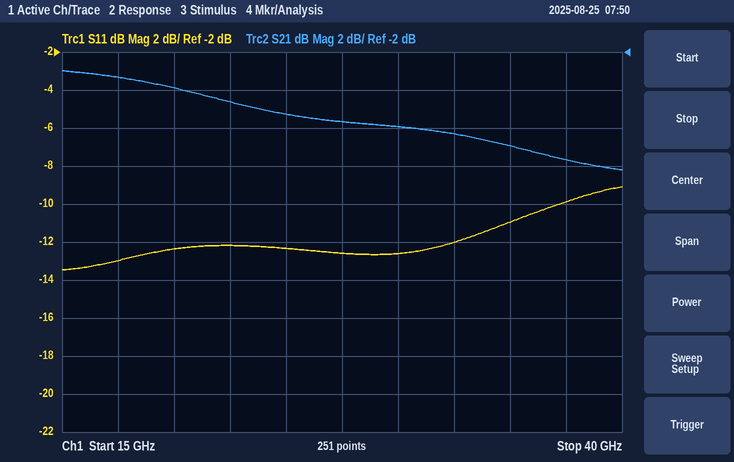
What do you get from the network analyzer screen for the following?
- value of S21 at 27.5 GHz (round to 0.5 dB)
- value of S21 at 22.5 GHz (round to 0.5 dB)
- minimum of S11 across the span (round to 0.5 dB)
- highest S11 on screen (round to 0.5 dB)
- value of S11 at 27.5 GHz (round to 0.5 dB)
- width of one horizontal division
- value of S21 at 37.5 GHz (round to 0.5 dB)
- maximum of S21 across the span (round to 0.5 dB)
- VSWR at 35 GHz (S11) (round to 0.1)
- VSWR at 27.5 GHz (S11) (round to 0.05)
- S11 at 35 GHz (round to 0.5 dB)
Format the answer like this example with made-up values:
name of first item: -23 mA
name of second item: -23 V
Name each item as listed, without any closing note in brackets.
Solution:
value of S21 at 27.5 GHz: -5.5 dB
value of S21 at 22.5 GHz: -4.5 dB
minimum of S11 across the span: -13.5 dB
highest S11 on screen: -9.0 dB
value of S11 at 27.5 GHz: -12.5 dB
width of one horizontal division: 2.5 GHz
value of S21 at 37.5 GHz: -7.5 dB
maximum of S21 across the span: -3.0 dB
VSWR at 35 GHz (S11): 1.8
VSWR at 27.5 GHz (S11): 1.60
S11 at 35 GHz: -11.0 dB
